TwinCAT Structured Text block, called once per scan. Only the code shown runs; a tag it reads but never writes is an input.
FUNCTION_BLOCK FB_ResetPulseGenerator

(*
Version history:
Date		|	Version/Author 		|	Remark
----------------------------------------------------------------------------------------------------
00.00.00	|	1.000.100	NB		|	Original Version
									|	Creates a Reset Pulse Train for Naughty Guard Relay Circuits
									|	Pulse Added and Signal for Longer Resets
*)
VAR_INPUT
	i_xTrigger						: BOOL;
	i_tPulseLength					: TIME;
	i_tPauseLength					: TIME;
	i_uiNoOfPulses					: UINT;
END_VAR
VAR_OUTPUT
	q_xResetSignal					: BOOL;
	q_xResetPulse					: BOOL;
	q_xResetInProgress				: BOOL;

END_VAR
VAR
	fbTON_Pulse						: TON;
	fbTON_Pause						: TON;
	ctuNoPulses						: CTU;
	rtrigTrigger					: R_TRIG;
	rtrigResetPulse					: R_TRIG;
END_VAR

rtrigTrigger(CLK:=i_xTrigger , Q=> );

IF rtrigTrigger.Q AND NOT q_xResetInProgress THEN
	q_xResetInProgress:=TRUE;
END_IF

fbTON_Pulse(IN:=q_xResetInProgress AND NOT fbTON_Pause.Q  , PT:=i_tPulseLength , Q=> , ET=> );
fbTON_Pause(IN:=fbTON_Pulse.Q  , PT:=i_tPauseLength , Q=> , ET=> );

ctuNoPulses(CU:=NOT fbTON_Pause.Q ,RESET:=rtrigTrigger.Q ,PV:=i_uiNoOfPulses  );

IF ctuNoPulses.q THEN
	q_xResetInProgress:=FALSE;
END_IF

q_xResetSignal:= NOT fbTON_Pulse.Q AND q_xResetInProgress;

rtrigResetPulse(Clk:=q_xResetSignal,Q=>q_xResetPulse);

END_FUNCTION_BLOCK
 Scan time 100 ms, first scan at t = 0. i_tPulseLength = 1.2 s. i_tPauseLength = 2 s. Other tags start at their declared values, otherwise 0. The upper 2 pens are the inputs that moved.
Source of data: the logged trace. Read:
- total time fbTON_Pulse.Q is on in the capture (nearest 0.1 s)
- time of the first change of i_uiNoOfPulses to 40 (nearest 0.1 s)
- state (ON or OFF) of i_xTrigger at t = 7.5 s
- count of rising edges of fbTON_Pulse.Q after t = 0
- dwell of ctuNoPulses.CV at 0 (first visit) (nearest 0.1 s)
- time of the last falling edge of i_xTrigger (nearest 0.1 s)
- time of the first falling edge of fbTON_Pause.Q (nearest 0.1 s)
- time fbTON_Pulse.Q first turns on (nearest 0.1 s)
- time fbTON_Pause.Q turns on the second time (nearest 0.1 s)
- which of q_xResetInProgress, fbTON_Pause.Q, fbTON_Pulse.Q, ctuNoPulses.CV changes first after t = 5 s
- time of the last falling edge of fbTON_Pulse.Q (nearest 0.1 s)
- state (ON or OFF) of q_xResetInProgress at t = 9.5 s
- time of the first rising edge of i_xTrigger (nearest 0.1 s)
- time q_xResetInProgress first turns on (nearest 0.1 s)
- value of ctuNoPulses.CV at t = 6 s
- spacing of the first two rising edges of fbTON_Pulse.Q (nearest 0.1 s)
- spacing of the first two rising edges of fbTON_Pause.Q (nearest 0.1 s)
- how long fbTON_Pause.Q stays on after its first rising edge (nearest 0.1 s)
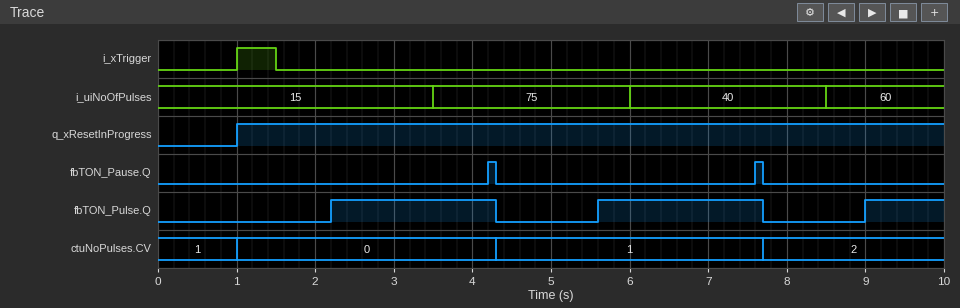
5.2 s
6.0 s
OFF
3
3.3 s
1.5 s
4.3 s
2.2 s
7.6 s
fbTON_Pulse.Q
7.7 s
ON
1.0 s
1.0 s
1
3.4 s
3.4 s
0.1 s
